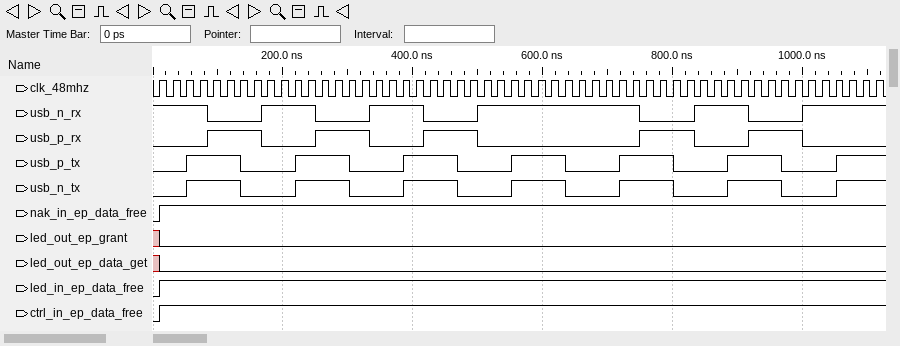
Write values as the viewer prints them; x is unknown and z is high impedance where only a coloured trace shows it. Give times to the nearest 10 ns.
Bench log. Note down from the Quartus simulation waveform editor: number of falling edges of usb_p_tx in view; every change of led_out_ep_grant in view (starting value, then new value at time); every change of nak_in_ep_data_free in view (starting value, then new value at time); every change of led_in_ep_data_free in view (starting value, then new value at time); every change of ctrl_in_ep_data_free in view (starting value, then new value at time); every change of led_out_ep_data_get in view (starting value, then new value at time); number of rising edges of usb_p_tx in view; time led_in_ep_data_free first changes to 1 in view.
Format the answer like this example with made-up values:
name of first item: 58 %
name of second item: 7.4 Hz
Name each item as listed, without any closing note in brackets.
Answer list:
number of falling edges of usb_p_tx in view: 6
every change of led_out_ep_grant in view: x, 0 at 10 ns
every change of nak_in_ep_data_free in view: 0, 1 at 10 ns
every change of led_in_ep_data_free in view: 0, 1 at 10 ns
every change of ctrl_in_ep_data_free in view: 0, 1 at 10 ns
every change of led_out_ep_data_get in view: x, 0 at 10 ns
number of rising edges of usb_p_tx in view: 7
time led_in_ep_data_free first changes to 1 in view: 10 ns
